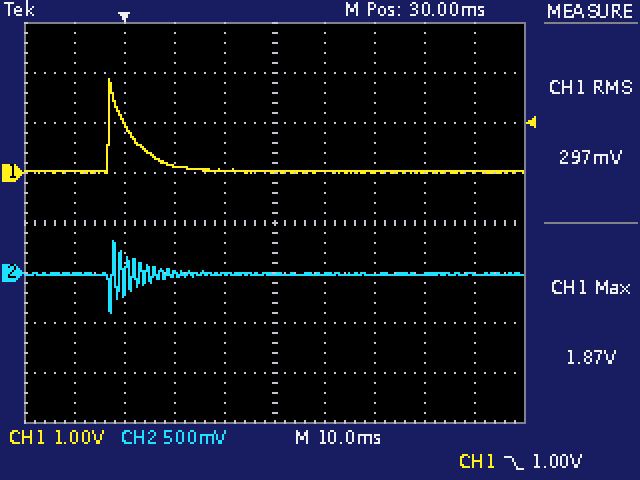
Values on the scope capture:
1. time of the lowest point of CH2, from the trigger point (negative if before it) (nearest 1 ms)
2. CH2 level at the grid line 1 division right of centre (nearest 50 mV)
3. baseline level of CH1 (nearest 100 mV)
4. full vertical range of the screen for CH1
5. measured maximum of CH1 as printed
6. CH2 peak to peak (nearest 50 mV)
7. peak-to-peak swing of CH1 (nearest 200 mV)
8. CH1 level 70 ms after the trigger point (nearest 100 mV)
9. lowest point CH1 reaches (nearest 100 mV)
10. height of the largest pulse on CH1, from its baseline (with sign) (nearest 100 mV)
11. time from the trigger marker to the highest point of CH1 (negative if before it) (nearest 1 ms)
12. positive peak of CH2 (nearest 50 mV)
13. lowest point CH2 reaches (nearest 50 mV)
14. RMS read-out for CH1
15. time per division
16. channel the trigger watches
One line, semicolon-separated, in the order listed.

-3 ms; 0 mV; 0.0 V; 8 V; 1.87 V; 700 mV; 1.8 V; 0.0 V; 0.0 V; +1.8 V; -3 ms; 300 mV; -400 mV; 297 mV; 10 ms; CH1
